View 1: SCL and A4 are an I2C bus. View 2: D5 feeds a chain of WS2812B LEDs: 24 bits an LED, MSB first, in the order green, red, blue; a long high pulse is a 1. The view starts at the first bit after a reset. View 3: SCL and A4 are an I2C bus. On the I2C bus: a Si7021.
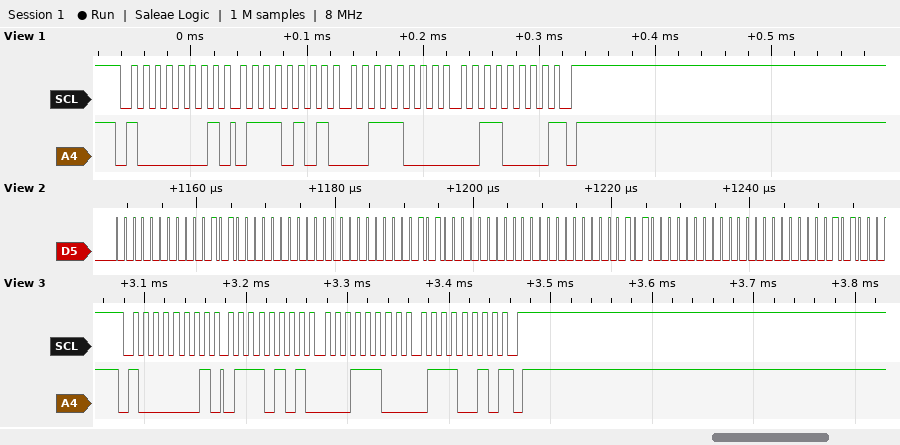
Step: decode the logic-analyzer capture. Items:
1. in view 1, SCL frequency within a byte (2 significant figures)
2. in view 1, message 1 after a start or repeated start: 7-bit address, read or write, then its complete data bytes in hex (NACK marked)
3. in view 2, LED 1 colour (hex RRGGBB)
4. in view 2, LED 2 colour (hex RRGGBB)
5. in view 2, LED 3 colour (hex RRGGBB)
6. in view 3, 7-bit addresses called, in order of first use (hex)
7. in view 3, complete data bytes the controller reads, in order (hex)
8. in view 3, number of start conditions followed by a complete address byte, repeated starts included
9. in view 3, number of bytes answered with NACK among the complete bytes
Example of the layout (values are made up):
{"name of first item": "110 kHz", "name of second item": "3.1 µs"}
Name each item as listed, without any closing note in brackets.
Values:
{"in view 1, SCL frequency within a byte": "100 kHz", "in view 1, message 1 after a start or repeated start: 7-bit address, read or write, then its complete data bytes in hex": "0x40 read: 75 38 30 NACK", "in view 2, LED 1 colour": "#140000", "in view 2, LED 2 colour": "#140000", "in view 2, LED 3 colour": "#140000", "in view 3, 7-bit addresses called, in order of first use": "0x40", "in view 3, complete data bytes the controller reads, in order": "75 1C 72", "in view 3, number of start conditions followed by a complete address byte, repeated starts included": "1", "in view 3, number of bytes answered with NACK among the complete bytes": "1"}
